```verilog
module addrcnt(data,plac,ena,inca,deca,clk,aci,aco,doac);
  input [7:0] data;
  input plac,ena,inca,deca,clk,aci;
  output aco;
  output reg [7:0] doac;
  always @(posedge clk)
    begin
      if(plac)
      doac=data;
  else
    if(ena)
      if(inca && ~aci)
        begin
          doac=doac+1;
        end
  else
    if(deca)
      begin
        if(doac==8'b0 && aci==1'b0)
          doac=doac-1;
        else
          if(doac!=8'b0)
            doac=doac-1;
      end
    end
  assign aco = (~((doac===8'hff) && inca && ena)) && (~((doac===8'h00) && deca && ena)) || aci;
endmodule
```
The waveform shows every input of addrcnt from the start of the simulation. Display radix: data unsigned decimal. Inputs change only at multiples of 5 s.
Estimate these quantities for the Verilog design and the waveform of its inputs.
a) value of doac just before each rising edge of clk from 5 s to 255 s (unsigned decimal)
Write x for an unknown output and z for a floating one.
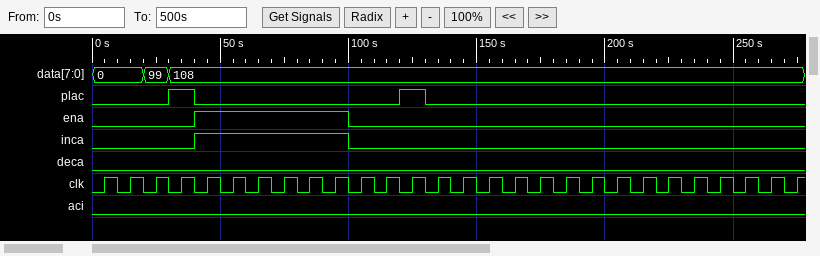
x, x, x, x, 108, 109, 110, 111, 112, 113, 114, 114, 114, 108, 108, 108, 108, 108, 108, 108, 108, 108, 108, 108, 108, 108
